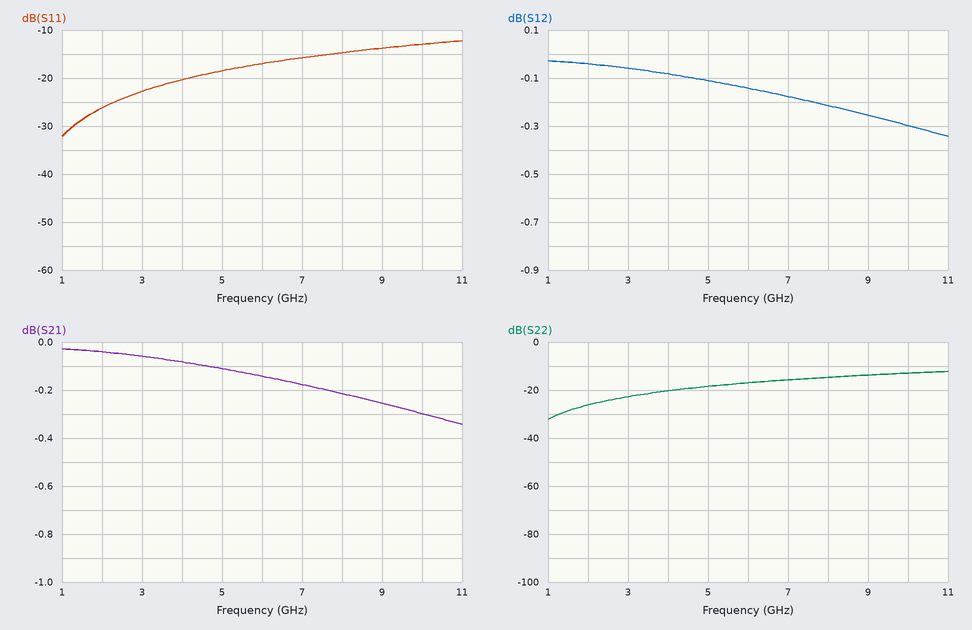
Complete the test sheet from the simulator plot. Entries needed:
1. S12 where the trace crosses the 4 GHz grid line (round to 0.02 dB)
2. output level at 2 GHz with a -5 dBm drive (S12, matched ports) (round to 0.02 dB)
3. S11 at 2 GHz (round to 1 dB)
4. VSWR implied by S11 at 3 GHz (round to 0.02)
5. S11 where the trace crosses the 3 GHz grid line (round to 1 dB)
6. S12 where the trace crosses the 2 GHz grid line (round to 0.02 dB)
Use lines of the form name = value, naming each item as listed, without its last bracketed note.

S12 where the trace crosses the 4 GHz grid line = -0.08 dB
output level at 2 GHz with a -5 dBm drive (S12, matched ports) = -5.04 dBm
S11 at 2 GHz = -26 dB
VSWR implied by S11 at 3 GHz = 1.16
S11 where the trace crosses the 3 GHz grid line = -23 dB
S12 where the trace crosses the 2 GHz grid line = -0.04 dB
